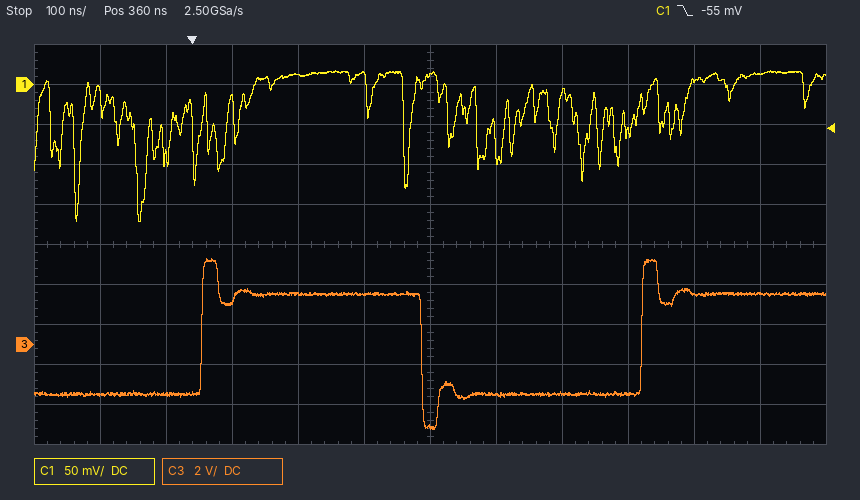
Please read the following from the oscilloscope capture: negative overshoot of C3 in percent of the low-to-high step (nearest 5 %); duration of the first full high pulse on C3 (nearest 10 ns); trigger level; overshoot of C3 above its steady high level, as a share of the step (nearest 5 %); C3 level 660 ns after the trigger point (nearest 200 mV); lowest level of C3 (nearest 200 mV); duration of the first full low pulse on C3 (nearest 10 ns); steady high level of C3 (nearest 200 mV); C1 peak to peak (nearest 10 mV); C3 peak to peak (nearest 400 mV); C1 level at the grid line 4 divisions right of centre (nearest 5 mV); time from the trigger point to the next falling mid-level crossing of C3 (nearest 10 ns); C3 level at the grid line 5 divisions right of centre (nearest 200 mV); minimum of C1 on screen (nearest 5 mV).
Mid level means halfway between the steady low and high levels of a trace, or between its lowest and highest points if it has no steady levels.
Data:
35 %
330 ns
-55 mV
35 %
-2.4 V
-4.2 V
330 ns
2.6 V
190 mV
8.4 V
5 mV
350 ns
2.6 V
-170 mV
